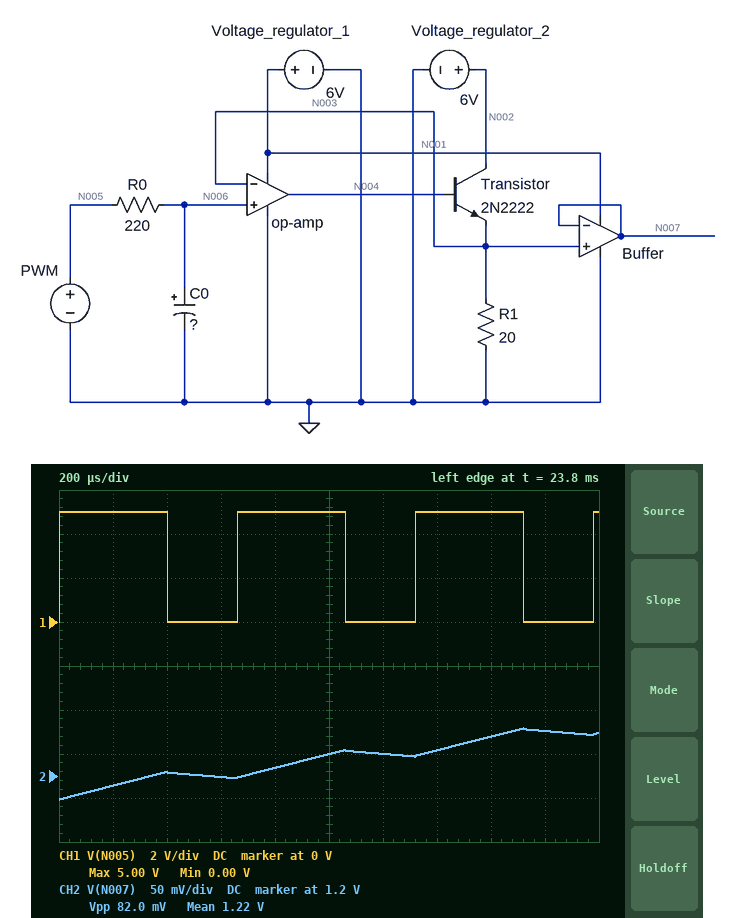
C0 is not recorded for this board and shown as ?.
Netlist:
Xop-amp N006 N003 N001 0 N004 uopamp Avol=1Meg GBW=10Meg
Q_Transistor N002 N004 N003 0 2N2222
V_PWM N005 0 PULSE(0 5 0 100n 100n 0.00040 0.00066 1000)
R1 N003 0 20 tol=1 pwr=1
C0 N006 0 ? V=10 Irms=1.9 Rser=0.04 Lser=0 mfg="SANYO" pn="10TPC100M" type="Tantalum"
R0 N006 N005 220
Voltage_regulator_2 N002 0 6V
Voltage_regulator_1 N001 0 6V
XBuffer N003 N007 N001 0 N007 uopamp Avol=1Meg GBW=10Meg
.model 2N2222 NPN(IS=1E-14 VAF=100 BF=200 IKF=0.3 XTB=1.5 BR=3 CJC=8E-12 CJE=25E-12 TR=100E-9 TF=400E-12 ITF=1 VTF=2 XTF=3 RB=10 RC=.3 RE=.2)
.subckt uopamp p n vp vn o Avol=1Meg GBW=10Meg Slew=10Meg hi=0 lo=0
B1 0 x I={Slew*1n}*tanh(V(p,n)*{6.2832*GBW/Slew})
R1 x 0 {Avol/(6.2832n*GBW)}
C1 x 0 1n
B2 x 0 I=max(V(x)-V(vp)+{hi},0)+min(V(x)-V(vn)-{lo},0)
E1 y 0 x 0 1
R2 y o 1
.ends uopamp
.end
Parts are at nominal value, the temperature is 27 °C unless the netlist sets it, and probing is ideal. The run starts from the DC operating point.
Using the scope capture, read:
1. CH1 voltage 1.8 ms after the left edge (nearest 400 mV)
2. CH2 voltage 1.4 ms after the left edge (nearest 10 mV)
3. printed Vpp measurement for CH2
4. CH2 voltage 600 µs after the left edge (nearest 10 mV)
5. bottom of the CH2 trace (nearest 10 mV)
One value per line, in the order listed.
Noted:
0 V
1.23 V
82.0 mV
1.20 V
1.17 V
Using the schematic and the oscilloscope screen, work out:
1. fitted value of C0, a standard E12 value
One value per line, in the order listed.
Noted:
220 µF
